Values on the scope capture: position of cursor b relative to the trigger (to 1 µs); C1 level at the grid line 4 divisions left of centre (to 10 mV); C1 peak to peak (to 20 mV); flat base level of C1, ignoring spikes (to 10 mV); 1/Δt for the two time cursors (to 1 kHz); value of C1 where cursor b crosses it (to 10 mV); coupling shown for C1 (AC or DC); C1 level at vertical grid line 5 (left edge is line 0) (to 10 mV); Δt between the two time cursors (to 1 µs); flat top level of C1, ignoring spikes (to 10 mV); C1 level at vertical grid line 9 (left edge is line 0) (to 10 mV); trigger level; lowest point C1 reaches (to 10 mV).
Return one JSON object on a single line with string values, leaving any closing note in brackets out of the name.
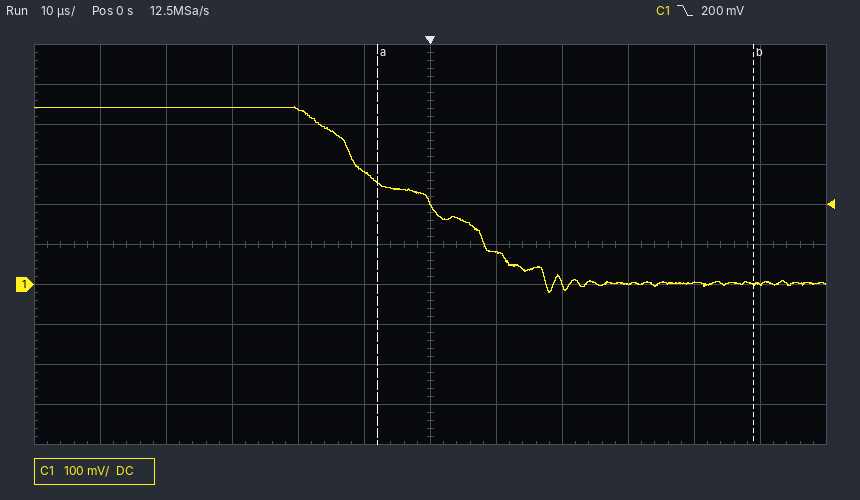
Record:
{"position of cursor b relative to the trigger": "+49 µs", "C1 level at the grid line 4 divisions left of centre": "440 mV", "C1 peak to peak": "460 mV", "flat base level of C1, ignoring spikes": "0 mV", "1/Δt for the two time cursors": "18 kHz", "value of C1 where cursor b crosses it": "0 mV", "coupling shown for C1": "DC", "C1 level at vertical grid line 5 (left edge is line 0)": "280 mV", "Δt between the two time cursors": "57 µs", "flat top level of C1, ignoring spikes": "440 mV", "C1 level at vertical grid line 9 (left edge is line 0)": "0 mV", "trigger level": "200 mV", "lowest point C1 reaches": "-20 mV"}
